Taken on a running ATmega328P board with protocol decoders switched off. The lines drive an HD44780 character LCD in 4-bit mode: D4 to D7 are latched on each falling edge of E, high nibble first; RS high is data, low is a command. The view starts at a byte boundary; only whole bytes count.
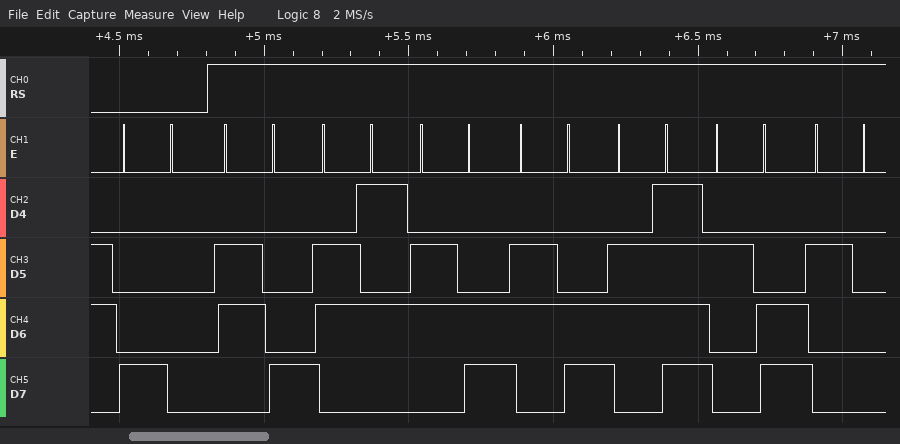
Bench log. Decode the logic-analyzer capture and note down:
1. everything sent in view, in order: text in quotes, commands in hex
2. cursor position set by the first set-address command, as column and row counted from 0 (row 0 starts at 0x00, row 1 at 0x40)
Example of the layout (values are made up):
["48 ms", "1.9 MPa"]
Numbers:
["0x80 \"hello, \"", "column 0, row 0"]
